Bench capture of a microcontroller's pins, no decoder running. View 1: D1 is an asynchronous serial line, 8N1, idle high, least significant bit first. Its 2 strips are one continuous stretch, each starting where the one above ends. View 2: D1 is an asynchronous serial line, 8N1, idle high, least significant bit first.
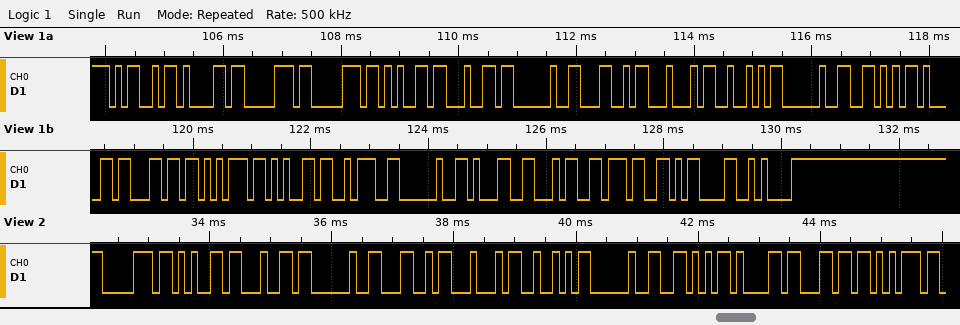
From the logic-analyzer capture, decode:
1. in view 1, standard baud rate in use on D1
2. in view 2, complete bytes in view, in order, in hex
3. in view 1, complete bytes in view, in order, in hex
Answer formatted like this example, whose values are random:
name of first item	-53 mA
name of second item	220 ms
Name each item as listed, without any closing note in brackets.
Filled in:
in view 1, standard baud rate in use on D1	9600 baud
in view 2, complete bytes in view, in order, in hex	0x70 0x65 0x64 0x20 0x4C 0x44 0x52 0x20 0x56 0x61 0x6C 0x75
in view 1, complete bytes in view, in order, in hex	4D 61 70 70 65 64 20 4C 44 52 20 56 61 6C 75 65 3A 20 31 34 37 0D 0A
